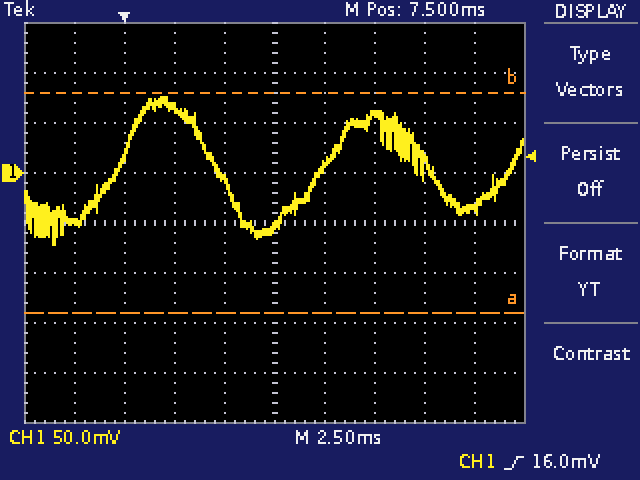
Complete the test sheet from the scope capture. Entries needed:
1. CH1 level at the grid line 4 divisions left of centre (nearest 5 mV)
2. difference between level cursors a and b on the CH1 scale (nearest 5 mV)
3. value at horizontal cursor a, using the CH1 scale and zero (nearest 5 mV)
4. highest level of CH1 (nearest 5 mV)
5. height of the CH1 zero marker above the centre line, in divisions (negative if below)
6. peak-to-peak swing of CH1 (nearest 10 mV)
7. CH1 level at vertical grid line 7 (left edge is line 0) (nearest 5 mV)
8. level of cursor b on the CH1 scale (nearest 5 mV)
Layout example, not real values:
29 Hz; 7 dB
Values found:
-50 mV; 220 mV; -140 mV; 75 mV; +1.0 div; 150 mV; 60 mV; 80 mV
